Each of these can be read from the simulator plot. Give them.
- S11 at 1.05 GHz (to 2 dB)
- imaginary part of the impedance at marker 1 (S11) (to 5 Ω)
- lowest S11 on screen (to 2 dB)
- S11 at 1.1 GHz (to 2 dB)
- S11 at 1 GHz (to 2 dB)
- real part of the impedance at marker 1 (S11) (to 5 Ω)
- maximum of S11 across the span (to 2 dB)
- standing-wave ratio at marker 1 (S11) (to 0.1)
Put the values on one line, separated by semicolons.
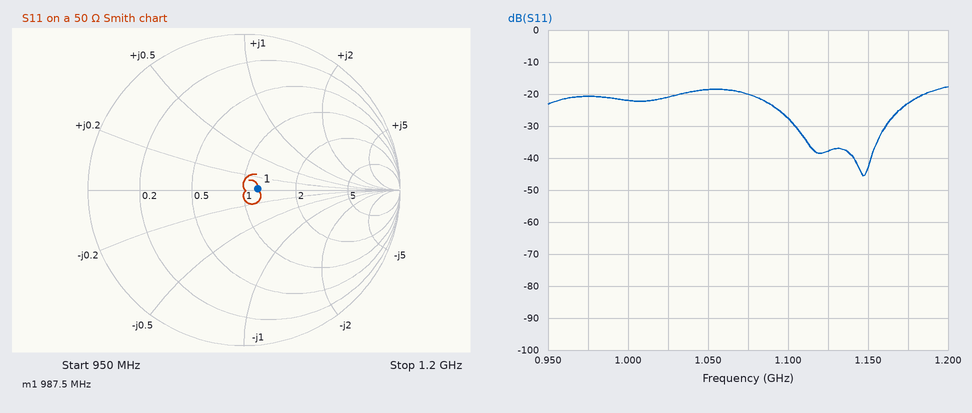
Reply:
-18 dB; 0 Ω; -46 dB; -28 dB; -22 dB; 60 Ω; -18 dB; 1.2
